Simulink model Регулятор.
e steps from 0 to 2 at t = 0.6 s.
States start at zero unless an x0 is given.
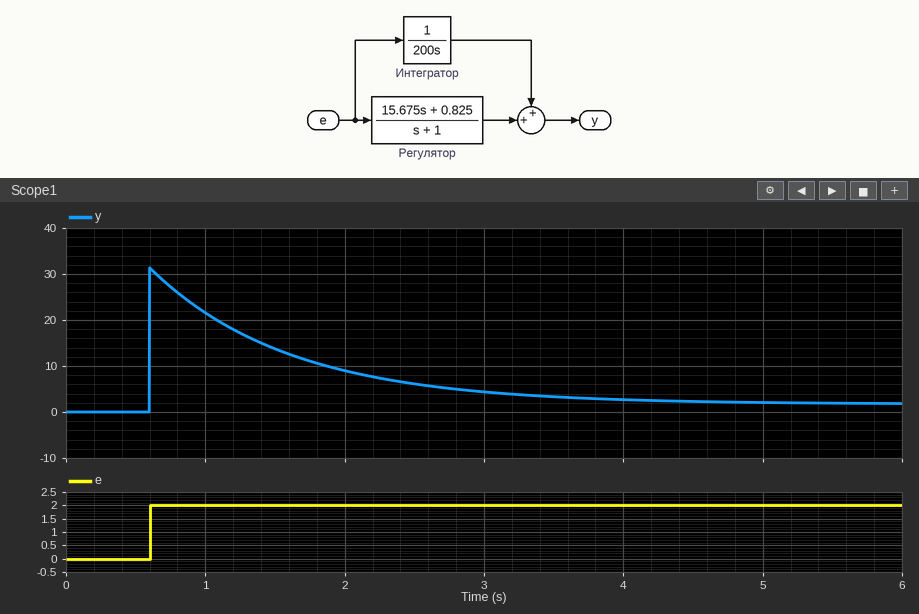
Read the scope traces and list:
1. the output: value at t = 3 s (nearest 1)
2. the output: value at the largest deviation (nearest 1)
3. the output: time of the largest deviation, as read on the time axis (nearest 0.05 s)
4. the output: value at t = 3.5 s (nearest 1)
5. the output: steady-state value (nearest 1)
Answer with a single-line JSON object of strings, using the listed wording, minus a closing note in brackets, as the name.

{"the output: value at t = 3 s": "4", "the output: value at the largest deviation": "31", "the output: time of the largest deviation, as read on the time axis": "0.60 s", "the output: value at t = 3.5 s": "3", "the output: steady-state value": "2"}
